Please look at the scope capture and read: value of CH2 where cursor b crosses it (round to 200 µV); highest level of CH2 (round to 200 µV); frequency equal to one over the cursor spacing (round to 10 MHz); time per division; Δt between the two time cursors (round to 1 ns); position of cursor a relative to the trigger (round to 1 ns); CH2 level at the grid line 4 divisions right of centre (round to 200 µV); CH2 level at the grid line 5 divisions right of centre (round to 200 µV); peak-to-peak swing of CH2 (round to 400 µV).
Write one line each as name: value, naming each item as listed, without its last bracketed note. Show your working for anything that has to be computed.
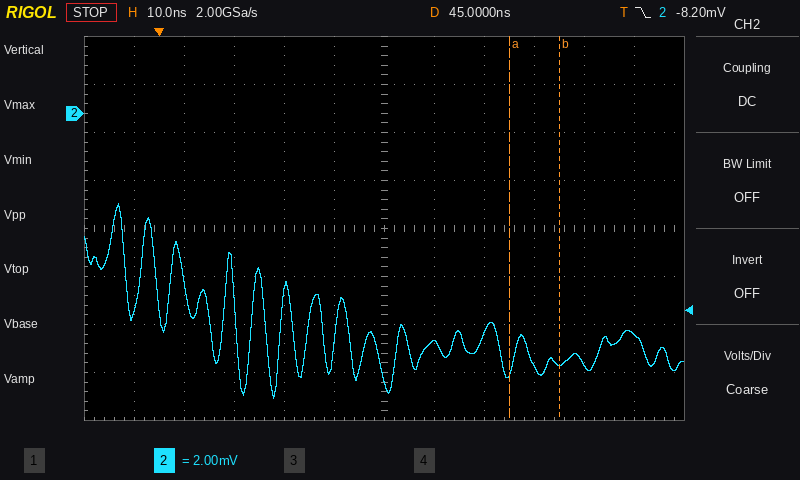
value of CH2 where cursor b crosses it: -10.4 mV
highest level of CH2: -3.8 mV
frequency equal to one over the cursor spacing: 1 / 10 ns ≈ 100 MHz
time per division: 10 ns
Δt between the two time cursors: 10 ns
position of cursor a relative to the trigger: +70 ns
CH2 level at the grid line 4 divisions right of centre: -10.4 mV
CH2 level at the grid line 5 divisions right of centre: -9.2 mV
peak-to-peak swing of CH2: 8.0 mV
